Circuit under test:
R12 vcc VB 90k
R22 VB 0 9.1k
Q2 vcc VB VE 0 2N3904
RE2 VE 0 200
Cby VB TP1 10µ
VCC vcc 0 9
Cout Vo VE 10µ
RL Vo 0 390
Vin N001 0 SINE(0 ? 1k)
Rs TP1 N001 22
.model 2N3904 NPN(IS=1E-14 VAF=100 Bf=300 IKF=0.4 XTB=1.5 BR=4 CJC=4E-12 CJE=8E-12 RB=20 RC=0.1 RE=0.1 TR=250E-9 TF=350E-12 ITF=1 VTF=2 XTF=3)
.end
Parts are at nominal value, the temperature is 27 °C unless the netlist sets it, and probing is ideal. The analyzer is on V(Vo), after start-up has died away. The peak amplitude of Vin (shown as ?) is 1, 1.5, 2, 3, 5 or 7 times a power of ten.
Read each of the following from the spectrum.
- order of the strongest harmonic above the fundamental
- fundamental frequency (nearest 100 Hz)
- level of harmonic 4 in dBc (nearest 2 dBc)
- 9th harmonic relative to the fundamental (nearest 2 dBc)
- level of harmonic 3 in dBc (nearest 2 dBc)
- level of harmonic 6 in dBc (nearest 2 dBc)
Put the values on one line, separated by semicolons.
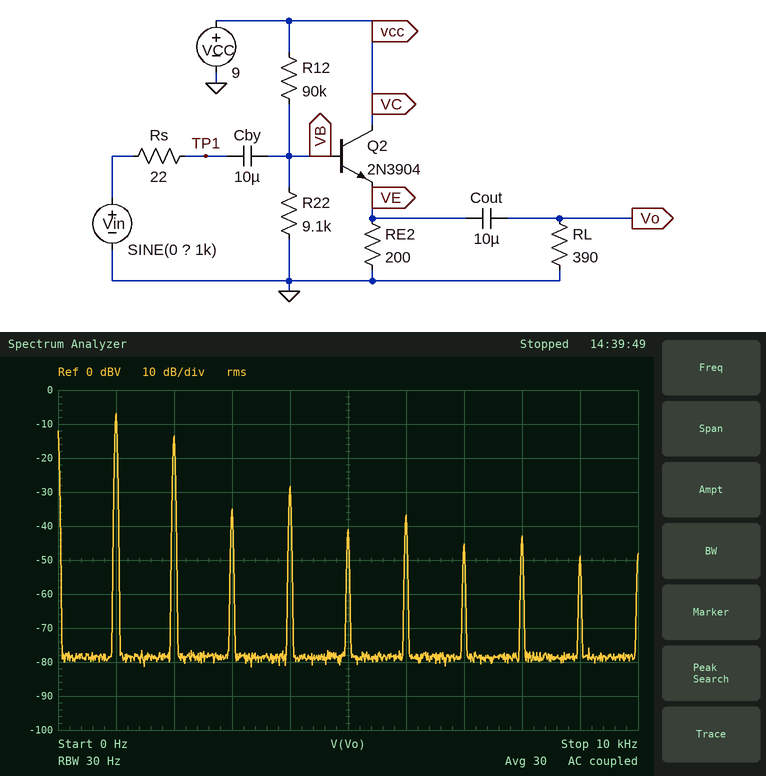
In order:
2; 1.0 kHz; -22 dBc; -42 dBc; -28 dBc; -30 dBc
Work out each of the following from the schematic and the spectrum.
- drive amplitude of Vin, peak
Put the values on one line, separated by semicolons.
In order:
1.5 V
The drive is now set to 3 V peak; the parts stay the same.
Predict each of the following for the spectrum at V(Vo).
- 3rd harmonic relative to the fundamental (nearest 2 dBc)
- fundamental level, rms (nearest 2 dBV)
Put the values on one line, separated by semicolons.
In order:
-24 dBc; -2 dBV
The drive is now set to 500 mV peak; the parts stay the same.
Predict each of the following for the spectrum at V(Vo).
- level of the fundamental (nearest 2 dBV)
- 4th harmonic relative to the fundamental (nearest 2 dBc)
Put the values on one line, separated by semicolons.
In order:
-14 dBV; -26 dBc
